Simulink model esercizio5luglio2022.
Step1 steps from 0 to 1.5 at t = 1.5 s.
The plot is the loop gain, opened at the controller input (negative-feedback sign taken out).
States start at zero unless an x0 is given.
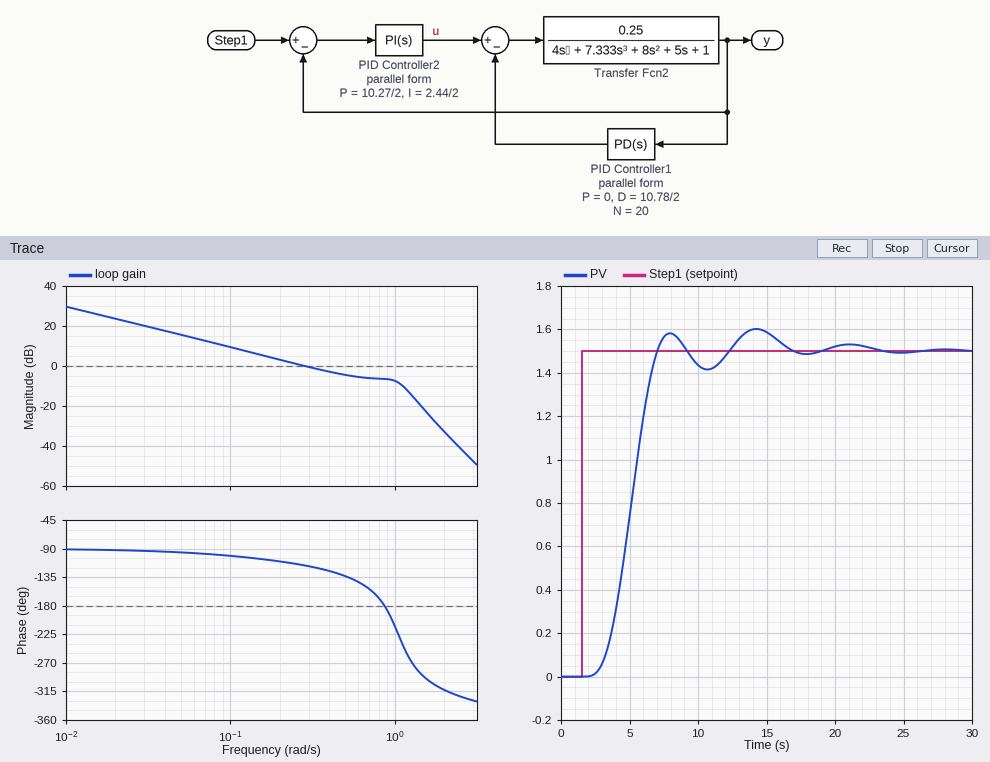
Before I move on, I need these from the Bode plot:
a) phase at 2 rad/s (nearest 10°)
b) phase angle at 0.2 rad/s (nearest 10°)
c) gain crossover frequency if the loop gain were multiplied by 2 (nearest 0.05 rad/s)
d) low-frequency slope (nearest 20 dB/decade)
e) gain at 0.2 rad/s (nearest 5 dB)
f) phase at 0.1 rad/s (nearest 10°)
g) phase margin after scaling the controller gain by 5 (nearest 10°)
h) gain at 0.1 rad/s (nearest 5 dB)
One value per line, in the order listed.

-310°
-110°
0.70 rad/s
-20 dB/decade
5 dB
-100°
-90°
10 dB
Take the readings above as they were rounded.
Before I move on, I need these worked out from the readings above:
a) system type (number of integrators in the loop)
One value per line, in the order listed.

1
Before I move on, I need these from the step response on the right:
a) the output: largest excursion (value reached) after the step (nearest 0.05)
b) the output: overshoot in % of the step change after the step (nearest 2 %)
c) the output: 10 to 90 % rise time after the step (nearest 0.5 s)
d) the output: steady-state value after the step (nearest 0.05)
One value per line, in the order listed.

1.60
6 %
3.0 s
1.50
